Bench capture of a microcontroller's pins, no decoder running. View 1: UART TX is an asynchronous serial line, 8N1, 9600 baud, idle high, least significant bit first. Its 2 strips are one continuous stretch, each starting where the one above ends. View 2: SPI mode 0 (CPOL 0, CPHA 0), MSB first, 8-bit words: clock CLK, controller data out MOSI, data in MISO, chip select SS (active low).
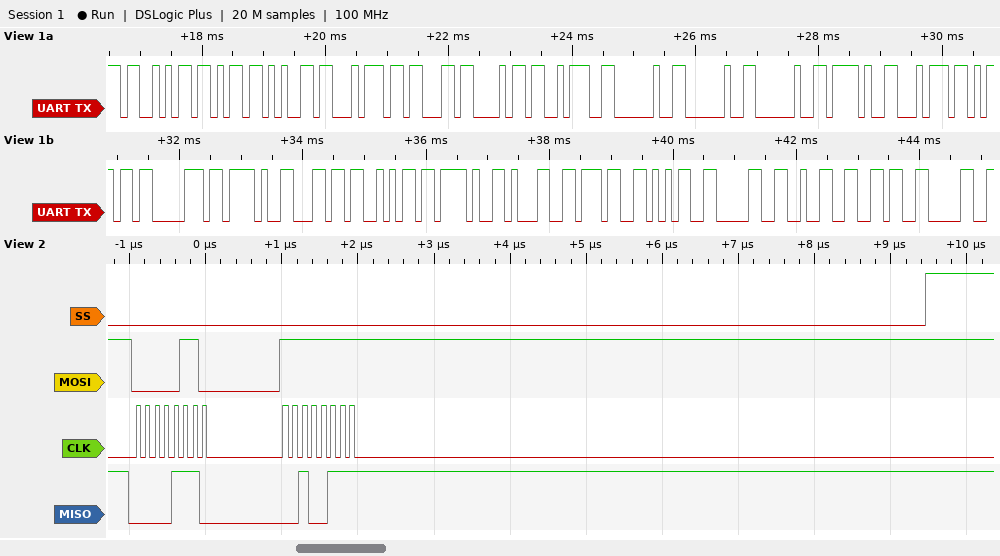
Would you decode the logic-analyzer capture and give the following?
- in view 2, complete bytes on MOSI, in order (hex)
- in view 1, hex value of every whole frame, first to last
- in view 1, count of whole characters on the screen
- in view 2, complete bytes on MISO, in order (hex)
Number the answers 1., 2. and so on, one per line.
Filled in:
1. 06 FF
2. 53 6B 65 74 63 68 3A 20 20 20 2F 74 6D 70 2F 6C 6A 2F 31 37 35 30 32 36 30
3. 25
4. 0E 27
